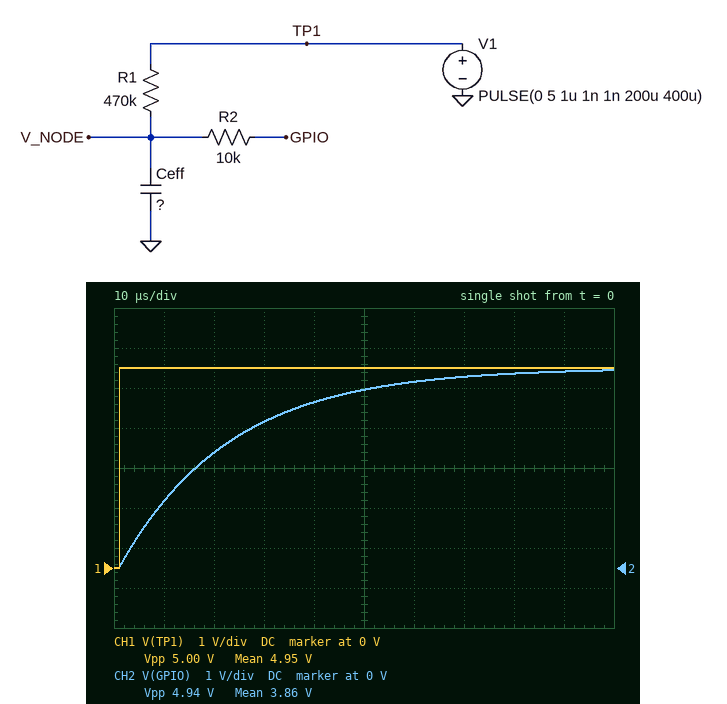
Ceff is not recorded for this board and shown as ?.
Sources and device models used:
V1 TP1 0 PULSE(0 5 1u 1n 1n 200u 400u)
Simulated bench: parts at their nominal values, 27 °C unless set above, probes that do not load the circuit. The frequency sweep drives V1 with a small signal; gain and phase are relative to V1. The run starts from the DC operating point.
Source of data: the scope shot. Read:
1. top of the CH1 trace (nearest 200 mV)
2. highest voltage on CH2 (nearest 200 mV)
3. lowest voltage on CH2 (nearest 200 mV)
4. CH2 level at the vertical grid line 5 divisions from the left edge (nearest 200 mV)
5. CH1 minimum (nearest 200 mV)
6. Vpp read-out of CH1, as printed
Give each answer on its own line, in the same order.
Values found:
5.0 V
5.0 V
0 V
4.4 V
0 V
5.00 V
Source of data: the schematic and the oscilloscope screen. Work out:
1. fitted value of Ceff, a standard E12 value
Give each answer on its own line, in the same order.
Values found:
47 pF
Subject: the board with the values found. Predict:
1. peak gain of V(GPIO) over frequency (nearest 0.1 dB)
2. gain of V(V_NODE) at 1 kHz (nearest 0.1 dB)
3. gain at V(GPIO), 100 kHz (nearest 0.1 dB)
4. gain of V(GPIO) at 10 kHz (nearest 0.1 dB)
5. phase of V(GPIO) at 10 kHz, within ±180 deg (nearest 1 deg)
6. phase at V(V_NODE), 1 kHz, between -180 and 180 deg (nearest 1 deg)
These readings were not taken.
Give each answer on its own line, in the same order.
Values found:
0 dB
-0.1 dB
-22.9 dB
-4.7 dB
-54 deg
-8 deg
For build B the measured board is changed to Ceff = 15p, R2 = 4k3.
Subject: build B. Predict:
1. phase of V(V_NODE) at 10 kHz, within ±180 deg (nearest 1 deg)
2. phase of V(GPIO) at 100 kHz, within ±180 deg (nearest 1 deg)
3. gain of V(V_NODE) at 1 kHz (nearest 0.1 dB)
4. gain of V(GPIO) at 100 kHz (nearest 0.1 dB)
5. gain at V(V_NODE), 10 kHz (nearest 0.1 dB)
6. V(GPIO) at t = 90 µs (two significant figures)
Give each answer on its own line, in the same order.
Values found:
-24 deg
-77 deg
0 dB
-13.1 dB
-0.8 dB
5.0 V
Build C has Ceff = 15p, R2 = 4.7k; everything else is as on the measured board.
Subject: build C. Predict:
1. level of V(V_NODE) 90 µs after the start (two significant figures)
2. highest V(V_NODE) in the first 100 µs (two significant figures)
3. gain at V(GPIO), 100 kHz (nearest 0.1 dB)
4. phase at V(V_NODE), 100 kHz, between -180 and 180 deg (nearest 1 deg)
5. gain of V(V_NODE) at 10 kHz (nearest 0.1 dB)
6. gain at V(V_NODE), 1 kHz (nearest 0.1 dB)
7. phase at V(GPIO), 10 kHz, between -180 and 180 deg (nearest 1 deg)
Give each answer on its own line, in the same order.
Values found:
5.0 V
5.0 V
-13.1 dB
-77 deg
-0.8 dB
0 dB
-24 deg
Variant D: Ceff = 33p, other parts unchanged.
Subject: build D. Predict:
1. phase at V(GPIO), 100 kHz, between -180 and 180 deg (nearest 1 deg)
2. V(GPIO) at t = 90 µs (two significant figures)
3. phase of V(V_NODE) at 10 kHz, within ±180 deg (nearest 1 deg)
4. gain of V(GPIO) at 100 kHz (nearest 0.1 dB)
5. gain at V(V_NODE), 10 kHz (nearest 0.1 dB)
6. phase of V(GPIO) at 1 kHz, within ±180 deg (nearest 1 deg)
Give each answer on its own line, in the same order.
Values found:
-84 deg
5.0 V
-44 deg
-19.8 dB
-2.9 dB
-6 deg
